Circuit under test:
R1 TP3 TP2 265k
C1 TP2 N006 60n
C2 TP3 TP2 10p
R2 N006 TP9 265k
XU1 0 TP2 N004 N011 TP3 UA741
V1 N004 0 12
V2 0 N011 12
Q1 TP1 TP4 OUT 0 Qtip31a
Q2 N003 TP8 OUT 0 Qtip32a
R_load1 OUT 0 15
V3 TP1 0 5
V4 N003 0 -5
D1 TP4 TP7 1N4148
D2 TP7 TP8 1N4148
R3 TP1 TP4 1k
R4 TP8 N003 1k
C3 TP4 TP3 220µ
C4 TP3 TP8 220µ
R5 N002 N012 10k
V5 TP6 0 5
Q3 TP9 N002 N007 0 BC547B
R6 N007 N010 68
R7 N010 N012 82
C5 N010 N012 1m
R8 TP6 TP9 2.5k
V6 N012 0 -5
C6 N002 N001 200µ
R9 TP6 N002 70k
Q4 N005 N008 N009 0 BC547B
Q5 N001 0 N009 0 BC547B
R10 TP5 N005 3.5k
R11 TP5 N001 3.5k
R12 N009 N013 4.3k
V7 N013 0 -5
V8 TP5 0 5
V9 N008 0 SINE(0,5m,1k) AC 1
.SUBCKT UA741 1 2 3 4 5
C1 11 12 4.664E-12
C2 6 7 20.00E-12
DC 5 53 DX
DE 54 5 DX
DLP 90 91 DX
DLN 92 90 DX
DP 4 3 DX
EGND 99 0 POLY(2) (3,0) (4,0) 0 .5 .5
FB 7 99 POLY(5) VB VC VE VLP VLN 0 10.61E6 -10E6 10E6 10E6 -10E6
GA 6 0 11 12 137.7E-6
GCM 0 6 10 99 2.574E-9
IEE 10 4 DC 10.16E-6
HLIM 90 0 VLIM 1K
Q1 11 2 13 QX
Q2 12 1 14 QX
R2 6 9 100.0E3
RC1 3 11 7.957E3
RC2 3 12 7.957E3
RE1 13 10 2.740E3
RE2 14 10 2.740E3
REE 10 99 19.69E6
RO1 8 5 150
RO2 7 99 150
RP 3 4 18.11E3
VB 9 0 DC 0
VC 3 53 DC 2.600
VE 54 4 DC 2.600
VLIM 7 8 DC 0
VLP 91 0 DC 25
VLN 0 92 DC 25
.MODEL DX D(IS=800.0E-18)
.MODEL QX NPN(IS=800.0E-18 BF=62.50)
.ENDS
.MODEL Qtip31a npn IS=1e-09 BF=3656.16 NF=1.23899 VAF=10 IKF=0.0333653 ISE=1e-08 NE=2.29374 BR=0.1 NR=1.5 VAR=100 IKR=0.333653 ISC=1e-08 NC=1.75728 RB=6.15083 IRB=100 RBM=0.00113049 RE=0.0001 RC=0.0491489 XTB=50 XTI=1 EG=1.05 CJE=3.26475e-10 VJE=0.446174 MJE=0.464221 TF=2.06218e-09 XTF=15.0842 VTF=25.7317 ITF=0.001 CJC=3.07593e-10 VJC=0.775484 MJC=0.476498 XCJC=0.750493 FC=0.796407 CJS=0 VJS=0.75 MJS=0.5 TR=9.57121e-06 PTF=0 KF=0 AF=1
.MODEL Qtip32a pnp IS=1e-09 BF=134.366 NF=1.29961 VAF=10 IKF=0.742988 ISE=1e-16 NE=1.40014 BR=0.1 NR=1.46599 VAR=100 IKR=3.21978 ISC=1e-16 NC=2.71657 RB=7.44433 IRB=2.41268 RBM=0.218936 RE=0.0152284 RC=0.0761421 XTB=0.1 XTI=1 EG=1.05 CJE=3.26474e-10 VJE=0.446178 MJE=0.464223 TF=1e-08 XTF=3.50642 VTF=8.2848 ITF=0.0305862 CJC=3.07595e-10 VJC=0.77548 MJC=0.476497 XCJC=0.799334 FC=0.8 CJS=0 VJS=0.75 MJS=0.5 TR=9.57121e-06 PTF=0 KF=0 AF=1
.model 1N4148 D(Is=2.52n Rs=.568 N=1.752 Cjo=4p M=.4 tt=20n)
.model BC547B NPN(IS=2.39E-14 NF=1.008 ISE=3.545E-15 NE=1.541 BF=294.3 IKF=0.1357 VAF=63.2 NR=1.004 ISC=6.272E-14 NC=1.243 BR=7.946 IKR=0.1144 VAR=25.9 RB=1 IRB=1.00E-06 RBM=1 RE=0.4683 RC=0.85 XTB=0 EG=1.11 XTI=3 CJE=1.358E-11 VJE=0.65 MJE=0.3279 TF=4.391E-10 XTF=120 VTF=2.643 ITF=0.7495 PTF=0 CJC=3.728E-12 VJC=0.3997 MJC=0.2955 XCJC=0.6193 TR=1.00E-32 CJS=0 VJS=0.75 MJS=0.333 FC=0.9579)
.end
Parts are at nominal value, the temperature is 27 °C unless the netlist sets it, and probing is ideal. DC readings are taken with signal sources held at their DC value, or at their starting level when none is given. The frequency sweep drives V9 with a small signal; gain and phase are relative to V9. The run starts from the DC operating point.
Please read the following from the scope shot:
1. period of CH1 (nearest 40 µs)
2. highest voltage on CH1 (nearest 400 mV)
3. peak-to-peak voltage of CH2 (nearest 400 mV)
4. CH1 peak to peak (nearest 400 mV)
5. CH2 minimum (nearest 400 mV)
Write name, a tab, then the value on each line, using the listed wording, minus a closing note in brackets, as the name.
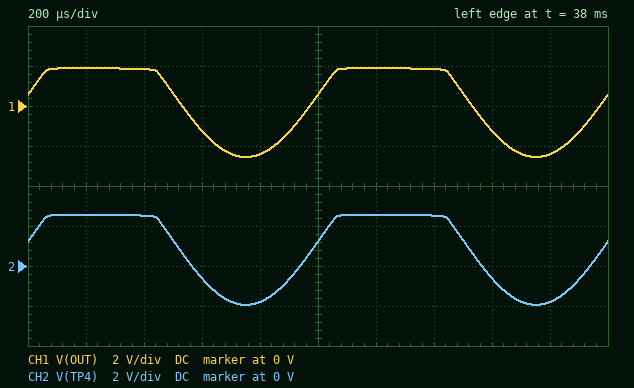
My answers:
period of CH1	1.00 ms
highest voltage on CH1	2.0 V
peak-to-peak voltage of CH2	4.4 V
CH1 peak to peak	4.4 V
CH2 minimum	-2.0 V
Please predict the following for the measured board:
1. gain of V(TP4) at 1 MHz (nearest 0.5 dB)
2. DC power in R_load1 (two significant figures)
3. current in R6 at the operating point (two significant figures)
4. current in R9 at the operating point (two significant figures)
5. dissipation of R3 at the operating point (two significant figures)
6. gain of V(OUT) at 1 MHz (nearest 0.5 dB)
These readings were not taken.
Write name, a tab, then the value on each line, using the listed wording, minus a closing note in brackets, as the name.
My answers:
gain of V(TP4) at 1 MHz	20.0 dB
DC power in R_load1	1.2 mW
current in R6 at the operating point	3.2 mA
current in R9 at the operating point	130 µA
dissipation of R3 at the operating point	18 mW
gain of V(OUT) at 1 MHz	20.0 dB
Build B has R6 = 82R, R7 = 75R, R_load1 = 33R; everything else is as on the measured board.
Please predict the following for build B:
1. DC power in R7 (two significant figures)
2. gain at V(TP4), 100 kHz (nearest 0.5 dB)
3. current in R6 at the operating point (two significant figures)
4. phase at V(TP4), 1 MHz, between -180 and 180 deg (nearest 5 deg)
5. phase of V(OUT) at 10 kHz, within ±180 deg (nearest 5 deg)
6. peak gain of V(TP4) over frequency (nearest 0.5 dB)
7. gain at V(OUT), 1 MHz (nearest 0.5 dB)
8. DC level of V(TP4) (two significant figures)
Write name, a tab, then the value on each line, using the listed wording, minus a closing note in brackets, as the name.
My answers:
DC power in R7	720 µW
gain at V(TP4), 100 kHz	48.5 dB
current in R6 at the operating point	3.1 mA
phase at V(TP4), 1 MHz, between -180 and 180 deg	90 deg
phase of V(OUT) at 10 kHz, within ±180 deg	-10 deg
peak gain of V(TP4) over frequency	55.0 dB
gain at V(OUT), 1 MHz	23.5 dB
DC level of V(TP4)	790 mV
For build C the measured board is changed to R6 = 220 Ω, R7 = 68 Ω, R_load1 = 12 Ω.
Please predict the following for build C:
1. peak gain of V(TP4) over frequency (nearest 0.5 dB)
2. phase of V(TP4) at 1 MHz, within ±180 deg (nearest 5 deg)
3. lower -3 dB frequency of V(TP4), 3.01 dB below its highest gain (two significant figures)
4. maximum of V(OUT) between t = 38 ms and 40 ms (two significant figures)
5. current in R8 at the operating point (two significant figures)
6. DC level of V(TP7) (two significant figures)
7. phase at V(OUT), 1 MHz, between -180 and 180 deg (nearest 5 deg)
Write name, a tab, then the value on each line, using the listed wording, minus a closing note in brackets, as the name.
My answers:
peak gain of V(TP4) over frequency	47.5 dB
phase of V(TP4) at 1 MHz, within ±180 deg	90 deg
lower -3 dB frequency of V(TP4), 3.01 dB below its highest gain	10 Hz
maximum of V(OUT) between t = 38 ms and 40 ms	1.3 V
current in R8 at the operating point	1.9 mA
DC level of V(TP7)	130 mV
phase at V(OUT), 1 MHz, between -180 and 180 deg	85 deg
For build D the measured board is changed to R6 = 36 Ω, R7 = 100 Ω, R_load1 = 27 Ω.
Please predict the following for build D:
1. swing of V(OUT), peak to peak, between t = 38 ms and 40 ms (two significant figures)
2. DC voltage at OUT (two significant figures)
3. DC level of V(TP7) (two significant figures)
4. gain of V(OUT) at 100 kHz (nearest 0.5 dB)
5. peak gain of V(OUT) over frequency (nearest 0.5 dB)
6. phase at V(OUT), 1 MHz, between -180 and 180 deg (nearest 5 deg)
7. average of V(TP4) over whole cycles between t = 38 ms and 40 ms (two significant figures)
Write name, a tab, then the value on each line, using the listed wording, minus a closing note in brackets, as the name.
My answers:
swing of V(OUT), peak to peak, between t = 38 ms and 40 ms	5.3 V
DC voltage at OUT	140 mV
DC level of V(TP7)	150 mV
gain of V(OUT) at 100 kHz	53.5 dB
peak gain of V(OUT) over frequency	60.0 dB
phase at V(OUT), 1 MHz, between -180 and 180 deg	65 deg
average of V(TP4) over whole cycles between t = 38 ms and 40 ms	840 mV
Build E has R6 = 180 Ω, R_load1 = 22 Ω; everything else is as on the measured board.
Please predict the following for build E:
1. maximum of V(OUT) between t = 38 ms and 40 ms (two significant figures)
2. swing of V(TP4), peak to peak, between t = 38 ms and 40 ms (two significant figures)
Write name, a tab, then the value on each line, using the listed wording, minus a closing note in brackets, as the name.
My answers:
maximum of V(OUT) between t = 38 ms and 40 ms	1.5 V
swing of V(TP4), peak to peak, between t = 38 ms and 40 ms	2.8 V
